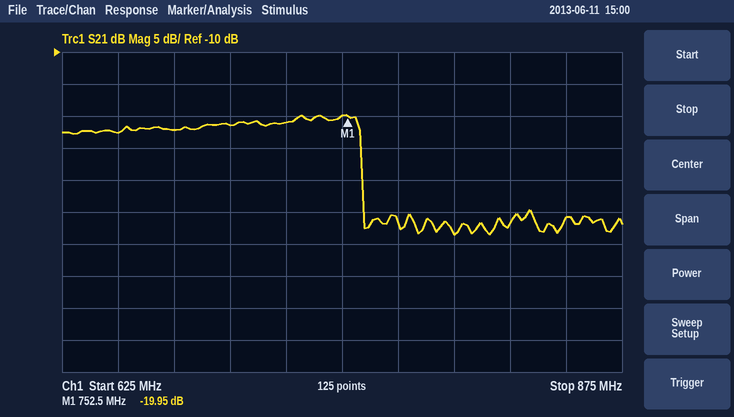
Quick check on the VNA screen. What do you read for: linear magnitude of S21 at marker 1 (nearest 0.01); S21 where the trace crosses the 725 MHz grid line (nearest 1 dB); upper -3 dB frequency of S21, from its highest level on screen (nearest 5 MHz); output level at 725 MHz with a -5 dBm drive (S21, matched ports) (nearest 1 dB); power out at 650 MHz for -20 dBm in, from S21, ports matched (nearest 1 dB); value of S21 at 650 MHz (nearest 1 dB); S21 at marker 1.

0.10
-21 dB
760 MHz
-26 dBm
-43 dBm
-23 dB
-19.95 dB
